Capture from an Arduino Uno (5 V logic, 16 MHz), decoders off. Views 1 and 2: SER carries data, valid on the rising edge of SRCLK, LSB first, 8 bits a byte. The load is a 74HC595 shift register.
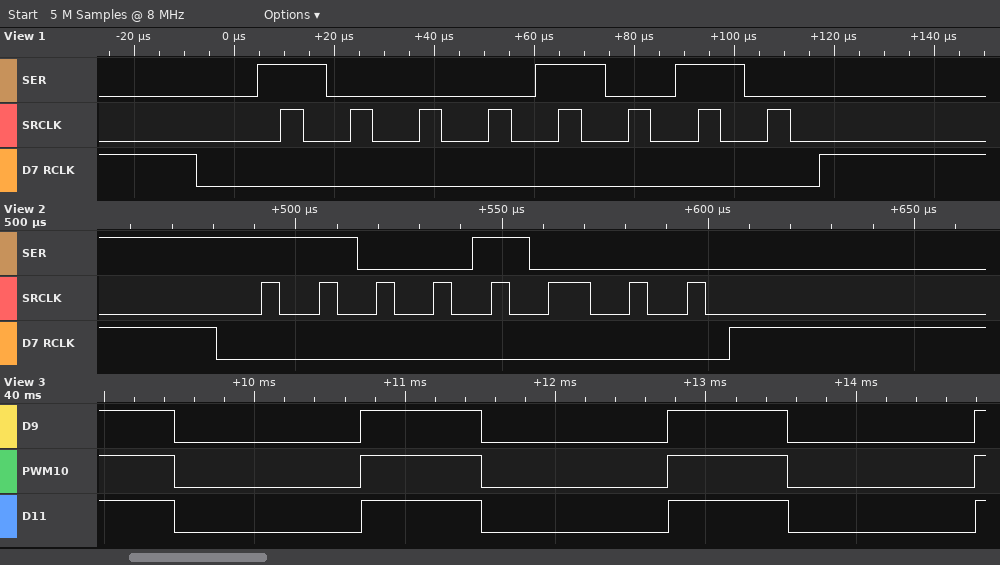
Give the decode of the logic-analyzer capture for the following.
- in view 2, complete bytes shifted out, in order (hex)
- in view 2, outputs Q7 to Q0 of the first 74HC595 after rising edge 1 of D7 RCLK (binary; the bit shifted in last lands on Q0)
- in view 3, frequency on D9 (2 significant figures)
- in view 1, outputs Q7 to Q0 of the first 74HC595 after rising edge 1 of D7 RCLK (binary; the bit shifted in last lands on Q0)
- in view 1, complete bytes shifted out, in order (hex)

0x13
11001000
490 Hz
10001010
51
